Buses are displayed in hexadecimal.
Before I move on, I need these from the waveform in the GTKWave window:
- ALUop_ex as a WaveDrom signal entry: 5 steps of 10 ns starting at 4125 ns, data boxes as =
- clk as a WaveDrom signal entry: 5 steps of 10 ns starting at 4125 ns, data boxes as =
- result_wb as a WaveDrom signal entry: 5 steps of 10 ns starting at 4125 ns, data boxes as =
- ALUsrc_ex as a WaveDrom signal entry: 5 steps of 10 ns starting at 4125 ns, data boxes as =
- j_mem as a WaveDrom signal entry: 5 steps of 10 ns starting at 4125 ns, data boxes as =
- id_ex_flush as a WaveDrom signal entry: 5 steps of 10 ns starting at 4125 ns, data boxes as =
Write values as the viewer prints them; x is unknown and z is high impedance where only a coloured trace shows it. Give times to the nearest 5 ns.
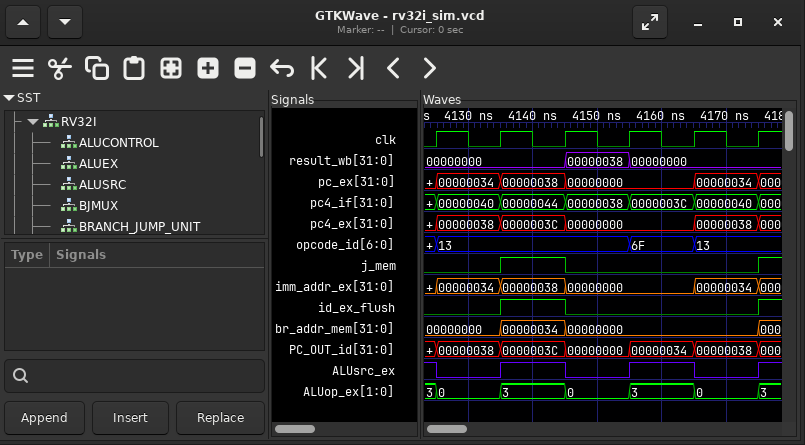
{name: 'ALUop_ex', wave: '=====', data: '0 3 0 3 0'}
{name: 'clk', wave: 'p....'}
{name: 'result_wb', wave: '=.==.', data: '00000000 00000038 00000000'}
{name: 'ALUsrc_ex', wave: '01010'}
{name: 'j_mem', wave: '010..'}
{name: 'id_ex_flush', wave: '010..'}
